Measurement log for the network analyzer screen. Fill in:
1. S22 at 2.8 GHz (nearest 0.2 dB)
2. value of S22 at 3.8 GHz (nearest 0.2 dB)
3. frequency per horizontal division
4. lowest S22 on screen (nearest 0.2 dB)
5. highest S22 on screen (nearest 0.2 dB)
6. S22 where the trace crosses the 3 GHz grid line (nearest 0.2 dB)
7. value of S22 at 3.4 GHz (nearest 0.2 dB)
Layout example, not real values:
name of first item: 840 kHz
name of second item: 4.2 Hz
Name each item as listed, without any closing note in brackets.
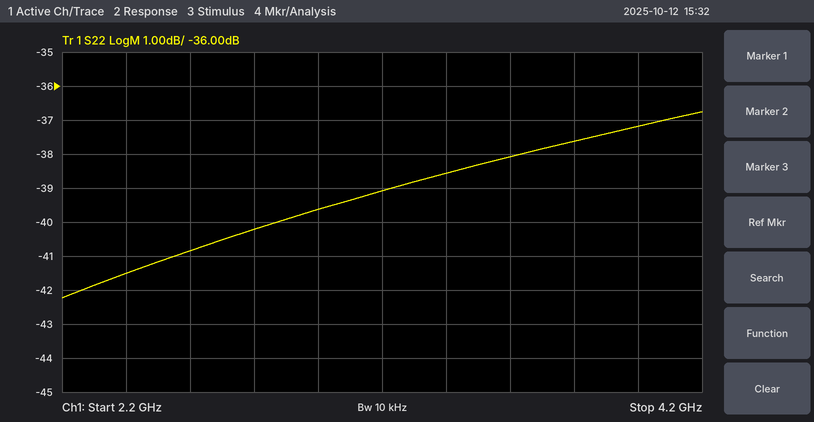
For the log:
S22 at 2.8 GHz: -40.2 dB
value of S22 at 3.8 GHz: -37.6 dB
frequency per horizontal division: 200 MHz
lowest S22 on screen: -42.2 dB
highest S22 on screen: -36.8 dB
S22 where the trace crosses the 3 GHz grid line: -39.6 dB
value of S22 at 3.4 GHz: -38.6 dB
